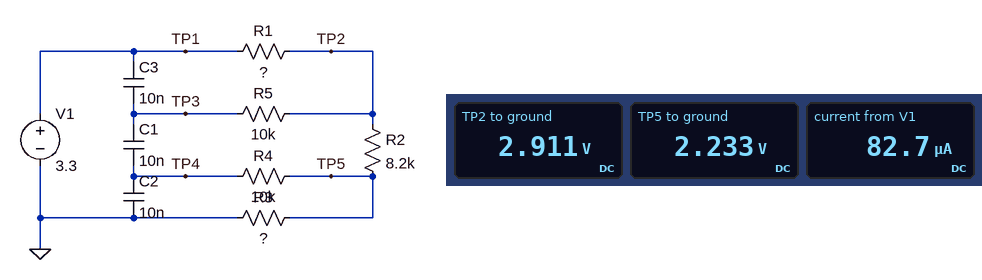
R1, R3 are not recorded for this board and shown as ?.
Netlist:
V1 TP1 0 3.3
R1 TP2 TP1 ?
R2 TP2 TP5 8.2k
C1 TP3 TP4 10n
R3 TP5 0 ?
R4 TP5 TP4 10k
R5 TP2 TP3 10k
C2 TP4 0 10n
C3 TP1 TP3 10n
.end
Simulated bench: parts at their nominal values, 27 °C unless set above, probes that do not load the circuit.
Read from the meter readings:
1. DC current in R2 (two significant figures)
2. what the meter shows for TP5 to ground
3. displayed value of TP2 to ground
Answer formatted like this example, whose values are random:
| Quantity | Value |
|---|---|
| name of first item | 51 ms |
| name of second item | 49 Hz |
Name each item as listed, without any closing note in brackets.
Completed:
| Quantity | Value |
|---|---|
| DC current in R2 | 83 µA |
| what the meter shows for TP5 to ground | 2.233 V |
| displayed value of TP2 to ground | 2.911 V |
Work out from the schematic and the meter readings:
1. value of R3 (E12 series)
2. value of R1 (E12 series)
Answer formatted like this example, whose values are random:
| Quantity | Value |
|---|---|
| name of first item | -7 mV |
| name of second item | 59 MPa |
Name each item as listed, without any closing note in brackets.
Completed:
| Quantity | Value |
|---|---|
| value of R3 | 27 kΩ |
| value of R1 | 4.7 kΩ |
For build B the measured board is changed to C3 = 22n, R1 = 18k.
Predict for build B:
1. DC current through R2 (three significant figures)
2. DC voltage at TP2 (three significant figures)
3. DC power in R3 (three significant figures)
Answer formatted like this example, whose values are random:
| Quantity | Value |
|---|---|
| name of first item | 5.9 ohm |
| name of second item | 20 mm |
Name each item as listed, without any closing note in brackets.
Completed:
| Quantity | Value |
|---|---|
| DC current through R2 | 62.0 µA |
| DC voltage at TP2 | 2.18 V |
| DC power in R3 | 104 µW |
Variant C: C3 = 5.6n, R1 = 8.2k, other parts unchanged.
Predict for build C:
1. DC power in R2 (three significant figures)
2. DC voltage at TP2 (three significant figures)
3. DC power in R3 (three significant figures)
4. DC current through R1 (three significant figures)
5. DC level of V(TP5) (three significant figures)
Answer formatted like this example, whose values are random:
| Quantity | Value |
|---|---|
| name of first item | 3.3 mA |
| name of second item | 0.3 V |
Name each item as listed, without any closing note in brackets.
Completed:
| Quantity | Value |
|---|---|
| DC power in R2 | 47.4 µW |
| DC voltage at TP2 | 2.68 V |
| DC power in R3 | 156 µW |
| DC current through R1 | 76.0 µA |
| DC level of V(TP5) | 2.05 V |
